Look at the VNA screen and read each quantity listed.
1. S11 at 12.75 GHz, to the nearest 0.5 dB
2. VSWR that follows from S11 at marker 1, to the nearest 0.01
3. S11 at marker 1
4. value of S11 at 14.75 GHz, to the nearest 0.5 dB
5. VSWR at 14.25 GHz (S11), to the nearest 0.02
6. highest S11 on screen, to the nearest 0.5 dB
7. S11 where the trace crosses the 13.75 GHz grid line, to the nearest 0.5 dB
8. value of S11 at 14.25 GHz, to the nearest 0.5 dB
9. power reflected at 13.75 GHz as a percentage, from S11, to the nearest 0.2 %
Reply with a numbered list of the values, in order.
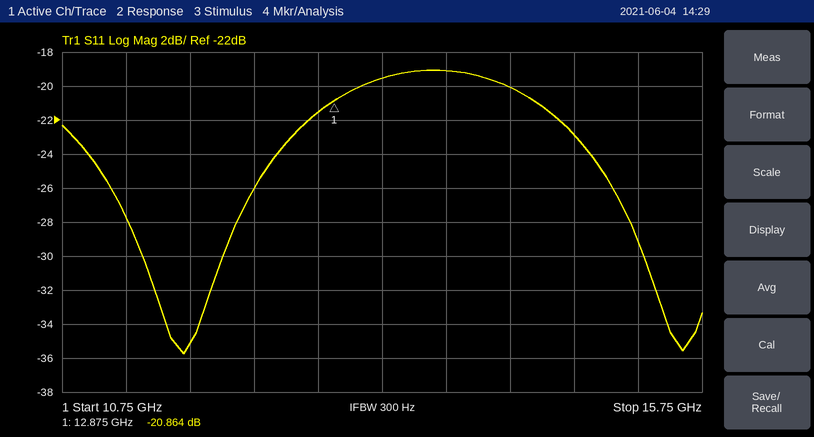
1. -21.5 dB
2. 1.20
3. -20.864 dB
4. -23.0 dB
5. 1.22
6. -19.0 dB
7. -19.0 dB
8. -20.0 dB
9. 1.2 %
